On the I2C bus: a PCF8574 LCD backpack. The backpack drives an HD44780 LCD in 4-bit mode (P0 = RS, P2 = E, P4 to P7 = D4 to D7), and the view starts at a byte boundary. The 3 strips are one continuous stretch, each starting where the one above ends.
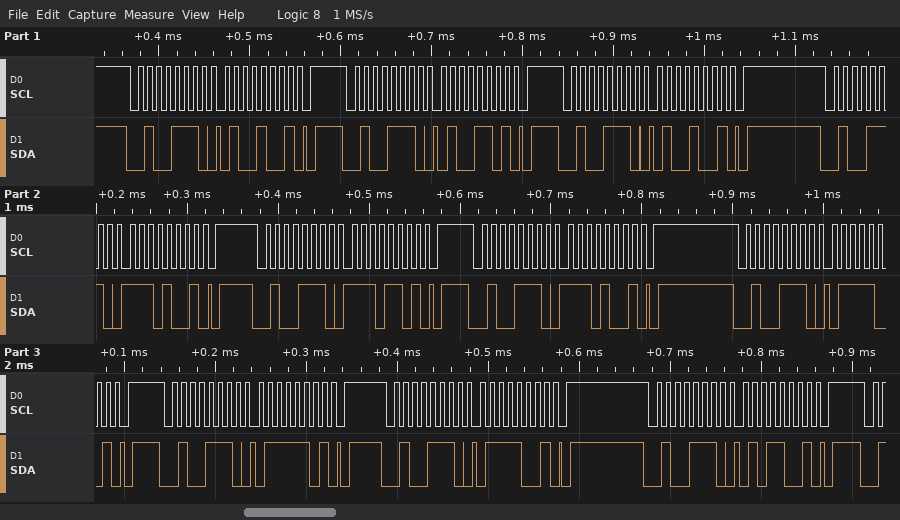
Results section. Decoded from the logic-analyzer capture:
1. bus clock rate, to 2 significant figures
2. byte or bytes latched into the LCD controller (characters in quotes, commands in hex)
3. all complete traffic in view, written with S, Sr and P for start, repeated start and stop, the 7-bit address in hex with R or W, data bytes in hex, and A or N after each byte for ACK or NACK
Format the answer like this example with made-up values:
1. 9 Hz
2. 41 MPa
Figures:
1. 100 kHz
2. 'N'
3. S 27W A 49 A P S 27W A 4D A P S 27W A 49 A P S 27W A E9 A P S 27W A ED A P S 27W A E9 A P S 27W A 79 A P S 27W A 7D A P S 27W A 79 A P S 27W A 59 A P
